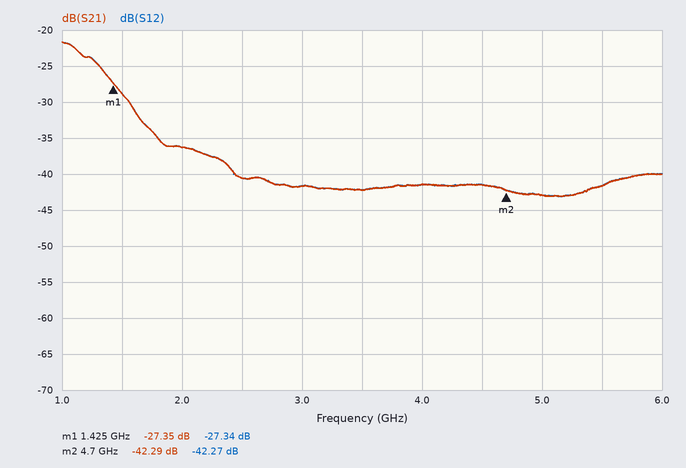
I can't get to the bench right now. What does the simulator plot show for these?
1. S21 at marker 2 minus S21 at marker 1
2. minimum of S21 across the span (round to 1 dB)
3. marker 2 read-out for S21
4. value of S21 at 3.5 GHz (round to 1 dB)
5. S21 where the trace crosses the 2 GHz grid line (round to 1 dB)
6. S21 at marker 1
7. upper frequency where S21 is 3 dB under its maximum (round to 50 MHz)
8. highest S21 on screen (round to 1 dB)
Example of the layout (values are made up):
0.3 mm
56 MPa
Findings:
-14.94 dB
-43 dB
-42.29 dB
-42 dB
-36 dB
-27.35 dB
1.30 GHz
-22 dB
